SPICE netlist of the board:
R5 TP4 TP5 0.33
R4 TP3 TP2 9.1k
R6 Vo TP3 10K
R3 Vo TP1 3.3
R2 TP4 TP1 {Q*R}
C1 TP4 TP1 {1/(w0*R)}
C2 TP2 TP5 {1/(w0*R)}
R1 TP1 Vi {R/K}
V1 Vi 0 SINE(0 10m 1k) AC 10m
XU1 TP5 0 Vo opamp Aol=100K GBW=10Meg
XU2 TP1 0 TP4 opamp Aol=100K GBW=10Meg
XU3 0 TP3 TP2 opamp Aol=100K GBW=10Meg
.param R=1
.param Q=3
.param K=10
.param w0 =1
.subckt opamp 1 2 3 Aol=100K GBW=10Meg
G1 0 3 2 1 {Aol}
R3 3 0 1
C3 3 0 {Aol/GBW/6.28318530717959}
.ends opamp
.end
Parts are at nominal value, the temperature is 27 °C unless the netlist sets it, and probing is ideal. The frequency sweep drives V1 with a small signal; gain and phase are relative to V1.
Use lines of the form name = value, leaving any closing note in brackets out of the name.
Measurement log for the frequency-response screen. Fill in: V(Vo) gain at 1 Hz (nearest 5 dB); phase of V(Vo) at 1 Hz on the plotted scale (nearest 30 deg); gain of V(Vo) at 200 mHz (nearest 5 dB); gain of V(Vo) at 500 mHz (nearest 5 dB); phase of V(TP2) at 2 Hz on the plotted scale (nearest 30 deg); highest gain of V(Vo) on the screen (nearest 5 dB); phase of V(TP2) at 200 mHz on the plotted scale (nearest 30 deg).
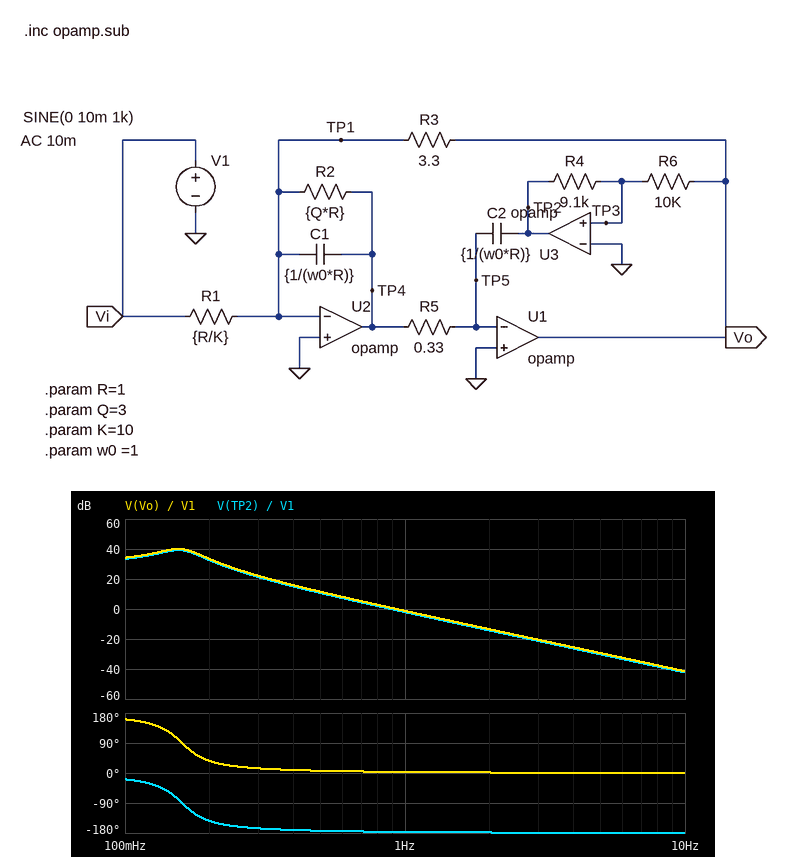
V(Vo) gain at 1 Hz = 0 dB
phase of V(Vo) at 1 Hz on the plotted scale = 0 deg
gain of V(Vo) at 200 mHz = 35 dB
gain of V(Vo) at 500 mHz = 10 dB
phase of V(TP2) at 2 Hz on the plotted scale = -180 deg
highest gain of V(Vo) on the screen = 40 dB
phase of V(TP2) at 200 mHz on the plotted scale = -150 deg
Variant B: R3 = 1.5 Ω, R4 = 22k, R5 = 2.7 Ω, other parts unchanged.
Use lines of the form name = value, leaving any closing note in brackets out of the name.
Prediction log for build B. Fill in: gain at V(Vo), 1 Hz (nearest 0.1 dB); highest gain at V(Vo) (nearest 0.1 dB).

gain at V(Vo), 1 Hz = -27.4 dB
highest gain at V(Vo) = 24.8 dB
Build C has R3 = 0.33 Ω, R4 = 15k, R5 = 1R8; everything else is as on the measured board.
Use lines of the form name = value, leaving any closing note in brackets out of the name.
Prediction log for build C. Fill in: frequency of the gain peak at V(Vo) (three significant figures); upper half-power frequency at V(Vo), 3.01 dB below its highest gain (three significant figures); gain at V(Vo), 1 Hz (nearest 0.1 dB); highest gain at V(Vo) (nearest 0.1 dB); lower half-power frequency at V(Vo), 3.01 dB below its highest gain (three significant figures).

frequency of the gain peak at V(Vo) = 164 mHz
upper half-power frequency at V(Vo), 3.01 dB below its highest gain = 189 mHz
gain at V(Vo), 1 Hz = -20.3 dB
highest gain at V(Vo) = 20.5 dB
lower half-power frequency at V(Vo), 3.01 dB below its highest gain = 135 mHz
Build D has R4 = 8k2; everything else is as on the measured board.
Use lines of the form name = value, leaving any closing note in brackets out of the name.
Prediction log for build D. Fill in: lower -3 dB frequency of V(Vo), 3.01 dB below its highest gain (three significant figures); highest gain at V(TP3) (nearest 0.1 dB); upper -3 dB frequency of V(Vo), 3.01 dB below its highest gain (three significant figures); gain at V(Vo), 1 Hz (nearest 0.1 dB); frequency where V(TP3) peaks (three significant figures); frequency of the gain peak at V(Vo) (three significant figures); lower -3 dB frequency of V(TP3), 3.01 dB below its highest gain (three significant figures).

lower -3 dB frequency of V(Vo), 3.01 dB below its highest gain = 135 mHz
highest gain at V(TP3) = -58.0 dB
upper -3 dB frequency of V(Vo), 3.01 dB below its highest gain = 189 mHz
gain at V(Vo), 1 Hz = -0.3 dB
frequency where V(TP3) peaks = 166 mHz
frequency of the gain peak at V(Vo) = 164 mHz
lower -3 dB frequency of V(TP3), 3.01 dB below its highest gain = 140 mHz
